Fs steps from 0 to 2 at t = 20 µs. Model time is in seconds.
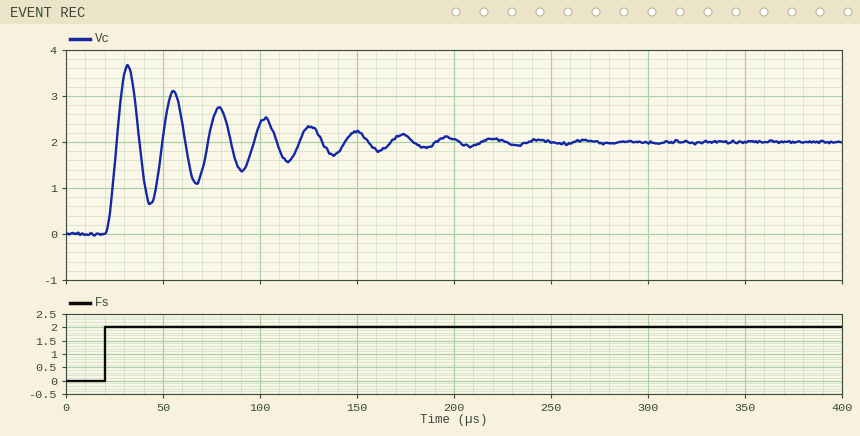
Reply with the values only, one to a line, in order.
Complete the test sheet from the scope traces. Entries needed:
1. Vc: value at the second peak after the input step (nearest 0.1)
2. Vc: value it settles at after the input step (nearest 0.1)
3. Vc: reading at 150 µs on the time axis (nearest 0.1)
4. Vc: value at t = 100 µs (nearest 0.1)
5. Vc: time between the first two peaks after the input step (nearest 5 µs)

3.1
2.0
2.2
2.4
25 µs
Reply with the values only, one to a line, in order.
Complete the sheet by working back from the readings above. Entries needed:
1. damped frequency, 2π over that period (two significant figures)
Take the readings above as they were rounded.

0.25 rad/µs
